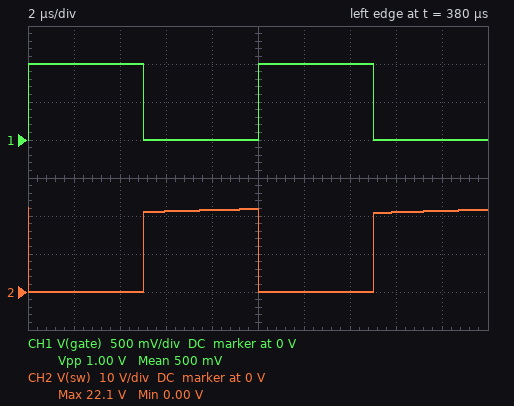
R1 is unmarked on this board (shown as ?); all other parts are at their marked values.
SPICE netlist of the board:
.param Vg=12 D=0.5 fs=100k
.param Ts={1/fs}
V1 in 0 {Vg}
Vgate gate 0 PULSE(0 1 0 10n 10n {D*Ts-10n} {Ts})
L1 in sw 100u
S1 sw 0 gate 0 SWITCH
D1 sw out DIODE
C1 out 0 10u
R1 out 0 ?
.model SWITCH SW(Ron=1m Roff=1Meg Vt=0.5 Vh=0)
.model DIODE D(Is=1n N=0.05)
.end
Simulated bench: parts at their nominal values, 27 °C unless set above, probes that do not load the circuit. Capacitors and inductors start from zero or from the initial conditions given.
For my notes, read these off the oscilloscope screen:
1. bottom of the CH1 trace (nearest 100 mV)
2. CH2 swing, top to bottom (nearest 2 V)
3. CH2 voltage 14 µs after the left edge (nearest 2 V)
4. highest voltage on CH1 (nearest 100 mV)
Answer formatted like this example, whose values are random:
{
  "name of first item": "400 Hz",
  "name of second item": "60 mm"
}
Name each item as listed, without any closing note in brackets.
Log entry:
{
  "bottom of the CH1 trace": "0 V",
  "CH2 swing, top to bottom": "22 V",
  "CH2 voltage 14 µs after the left edge": "0 V",
  "highest voltage on CH1": "1.0 V"
}
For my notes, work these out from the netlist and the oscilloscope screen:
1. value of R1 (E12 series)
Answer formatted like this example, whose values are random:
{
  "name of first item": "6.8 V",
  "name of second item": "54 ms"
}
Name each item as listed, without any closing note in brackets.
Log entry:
{
  "value of R1": "10 Ω"
}
